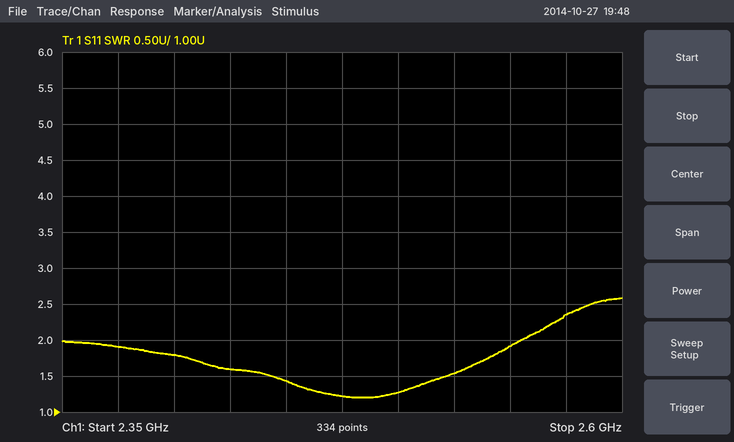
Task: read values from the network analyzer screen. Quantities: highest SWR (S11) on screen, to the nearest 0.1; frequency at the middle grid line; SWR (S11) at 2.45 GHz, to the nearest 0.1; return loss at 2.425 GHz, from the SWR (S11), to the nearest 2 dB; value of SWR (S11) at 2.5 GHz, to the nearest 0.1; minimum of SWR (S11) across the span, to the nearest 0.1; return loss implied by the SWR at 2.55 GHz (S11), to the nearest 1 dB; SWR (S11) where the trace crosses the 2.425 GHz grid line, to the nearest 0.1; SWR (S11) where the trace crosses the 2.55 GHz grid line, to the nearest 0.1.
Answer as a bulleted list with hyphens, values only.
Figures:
- 2.6
- 2.475 GHz
- 1.4
- 12 dB
- 1.3
- 1.2
- 10 dB
- 1.6
- 1.9
